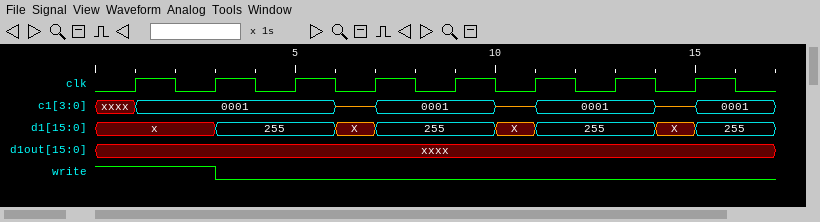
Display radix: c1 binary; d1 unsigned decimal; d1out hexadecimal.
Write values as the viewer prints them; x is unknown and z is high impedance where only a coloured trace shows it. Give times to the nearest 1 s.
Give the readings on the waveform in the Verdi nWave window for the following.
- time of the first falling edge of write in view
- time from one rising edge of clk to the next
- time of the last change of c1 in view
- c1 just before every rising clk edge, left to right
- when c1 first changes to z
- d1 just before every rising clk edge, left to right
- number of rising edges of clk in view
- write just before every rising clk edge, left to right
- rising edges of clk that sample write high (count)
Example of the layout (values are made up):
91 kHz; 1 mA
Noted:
3 s; 2 s; 15 s; xxxx, 0001, 0001, z, 0001, z, 0001, z; 6 s; x, x, 255, X, 255, X, 255, X; 8; 1 1 0 0 0 0 0 0; 2
